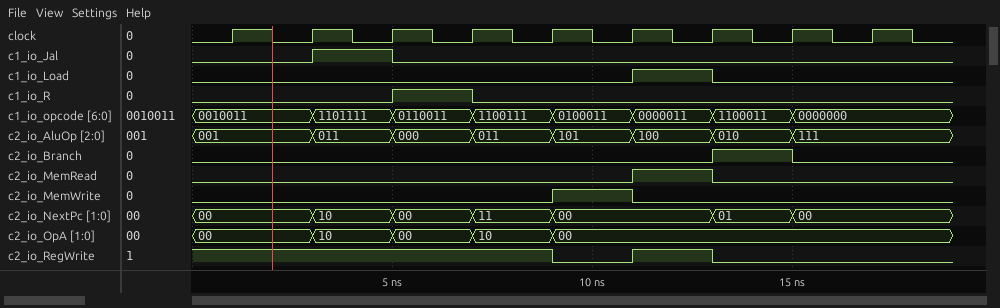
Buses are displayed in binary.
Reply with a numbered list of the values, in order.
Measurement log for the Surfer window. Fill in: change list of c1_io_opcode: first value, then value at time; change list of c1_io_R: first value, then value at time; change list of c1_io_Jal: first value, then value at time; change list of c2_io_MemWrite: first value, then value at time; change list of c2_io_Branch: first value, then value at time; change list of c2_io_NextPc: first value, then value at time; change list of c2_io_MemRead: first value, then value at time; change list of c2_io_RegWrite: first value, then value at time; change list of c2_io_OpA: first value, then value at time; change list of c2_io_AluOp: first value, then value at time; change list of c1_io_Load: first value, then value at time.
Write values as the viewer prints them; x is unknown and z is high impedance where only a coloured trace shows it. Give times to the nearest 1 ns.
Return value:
1. 0010011, 1101111 at 3 ns, 0110011 at 5 ns, 1100111 at 7 ns, 0100011 at 9 ns, 0000011 at 11 ns, 1100011 at 13 ns, 0000000 at 15 ns
2. 0, 1 at 5 ns, 0 at 7 ns
3. 0, 1 at 3 ns, 0 at 5 ns
4. 0, 1 at 9 ns, 0 at 11 ns
5. 0, 1 at 13 ns, 0 at 15 ns
6. 00, 10 at 3 ns, 00 at 5 ns, 11 at 7 ns, 00 at 9 ns, 01 at 13 ns, 00 at 15 ns
7. 0, 1 at 11 ns, 0 at 13 ns
8. 1, 0 at 9 ns, 1 at 11 ns, 0 at 13 ns
9. 00, 10 at 3 ns, 00 at 5 ns, 10 at 7 ns, 00 at 9 ns
10. 001, 011 at 3 ns, 000 at 5 ns, 011 at 7 ns, 101 at 9 ns, 100 at 11 ns, 010 at 13 ns, 111 at 15 ns
11. 0, 1 at 11 ns, 0 at 13 ns
